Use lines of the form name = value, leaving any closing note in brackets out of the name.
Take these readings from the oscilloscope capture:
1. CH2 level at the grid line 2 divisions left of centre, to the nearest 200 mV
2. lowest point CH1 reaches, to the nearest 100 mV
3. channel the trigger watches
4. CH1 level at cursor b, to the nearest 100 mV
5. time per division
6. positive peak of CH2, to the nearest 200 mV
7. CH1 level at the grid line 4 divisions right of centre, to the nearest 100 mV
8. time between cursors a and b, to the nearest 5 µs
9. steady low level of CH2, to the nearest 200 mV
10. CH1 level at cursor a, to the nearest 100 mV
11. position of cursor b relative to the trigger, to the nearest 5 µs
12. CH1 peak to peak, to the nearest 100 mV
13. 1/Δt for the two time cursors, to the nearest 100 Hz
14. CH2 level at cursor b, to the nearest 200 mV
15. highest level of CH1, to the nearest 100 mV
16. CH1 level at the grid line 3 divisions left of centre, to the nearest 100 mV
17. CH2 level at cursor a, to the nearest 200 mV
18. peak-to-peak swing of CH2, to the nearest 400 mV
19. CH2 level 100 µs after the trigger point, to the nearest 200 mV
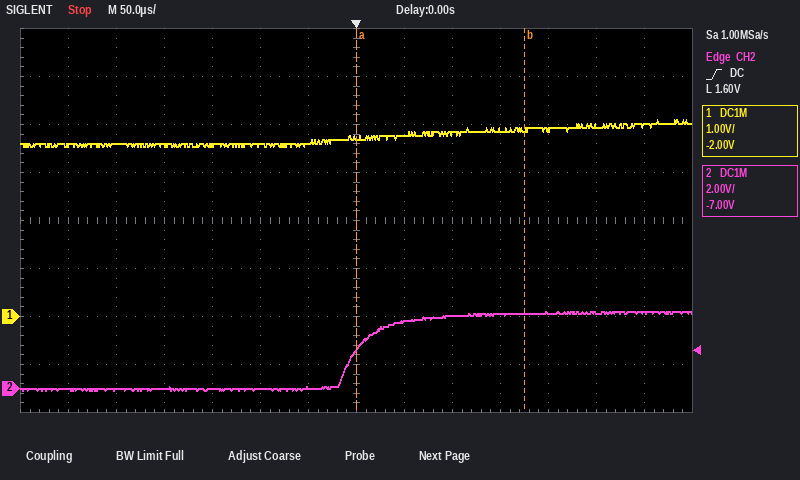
CH2 level at the grid line 2 divisions left of centre, to the nearest 200 mV = 0.0 V
lowest point CH1 reaches, to the nearest 100 mV = 3.5 V
channel the trigger watches = CH2
CH1 level at cursor b, to the nearest 100 mV = 3.9 V
time per division = 50 µs
positive peak of CH2, to the nearest 200 mV = 3.2 V
CH1 level at the grid line 4 divisions right of centre, to the nearest 100 mV = 3.9 V
time between cursors a and b, to the nearest 5 µs = 175 µs
steady low level of CH2, to the nearest 200 mV = 0.0 V
CH1 level at cursor a, to the nearest 100 mV = 3.7 V
position of cursor b relative to the trigger, to the nearest 5 µs = +175 µs
CH1 peak to peak, to the nearest 100 mV = 600 mV
1/Δt for the two time cursors, to the nearest 100 Hz = 5.7 kHz
CH2 level at cursor b, to the nearest 200 mV = 3.2 V
highest level of CH1, to the nearest 100 mV = 4.1 V
CH1 level at the grid line 3 divisions left of centre, to the nearest 100 mV = 3.6 V
CH2 level at cursor a, to the nearest 200 mV = 1.6 V
peak-to-peak swing of CH2, to the nearest 400 mV = 3.2 V
CH2 level 100 µs after the trigger point, to the nearest 200 mV = 3.0 V
